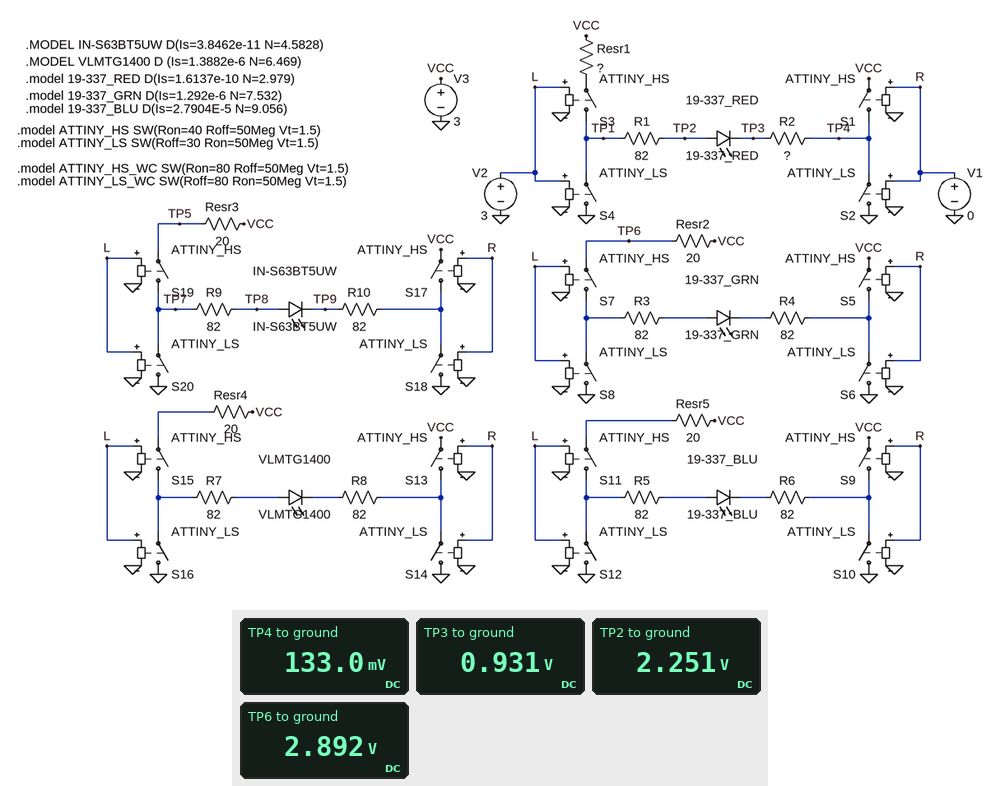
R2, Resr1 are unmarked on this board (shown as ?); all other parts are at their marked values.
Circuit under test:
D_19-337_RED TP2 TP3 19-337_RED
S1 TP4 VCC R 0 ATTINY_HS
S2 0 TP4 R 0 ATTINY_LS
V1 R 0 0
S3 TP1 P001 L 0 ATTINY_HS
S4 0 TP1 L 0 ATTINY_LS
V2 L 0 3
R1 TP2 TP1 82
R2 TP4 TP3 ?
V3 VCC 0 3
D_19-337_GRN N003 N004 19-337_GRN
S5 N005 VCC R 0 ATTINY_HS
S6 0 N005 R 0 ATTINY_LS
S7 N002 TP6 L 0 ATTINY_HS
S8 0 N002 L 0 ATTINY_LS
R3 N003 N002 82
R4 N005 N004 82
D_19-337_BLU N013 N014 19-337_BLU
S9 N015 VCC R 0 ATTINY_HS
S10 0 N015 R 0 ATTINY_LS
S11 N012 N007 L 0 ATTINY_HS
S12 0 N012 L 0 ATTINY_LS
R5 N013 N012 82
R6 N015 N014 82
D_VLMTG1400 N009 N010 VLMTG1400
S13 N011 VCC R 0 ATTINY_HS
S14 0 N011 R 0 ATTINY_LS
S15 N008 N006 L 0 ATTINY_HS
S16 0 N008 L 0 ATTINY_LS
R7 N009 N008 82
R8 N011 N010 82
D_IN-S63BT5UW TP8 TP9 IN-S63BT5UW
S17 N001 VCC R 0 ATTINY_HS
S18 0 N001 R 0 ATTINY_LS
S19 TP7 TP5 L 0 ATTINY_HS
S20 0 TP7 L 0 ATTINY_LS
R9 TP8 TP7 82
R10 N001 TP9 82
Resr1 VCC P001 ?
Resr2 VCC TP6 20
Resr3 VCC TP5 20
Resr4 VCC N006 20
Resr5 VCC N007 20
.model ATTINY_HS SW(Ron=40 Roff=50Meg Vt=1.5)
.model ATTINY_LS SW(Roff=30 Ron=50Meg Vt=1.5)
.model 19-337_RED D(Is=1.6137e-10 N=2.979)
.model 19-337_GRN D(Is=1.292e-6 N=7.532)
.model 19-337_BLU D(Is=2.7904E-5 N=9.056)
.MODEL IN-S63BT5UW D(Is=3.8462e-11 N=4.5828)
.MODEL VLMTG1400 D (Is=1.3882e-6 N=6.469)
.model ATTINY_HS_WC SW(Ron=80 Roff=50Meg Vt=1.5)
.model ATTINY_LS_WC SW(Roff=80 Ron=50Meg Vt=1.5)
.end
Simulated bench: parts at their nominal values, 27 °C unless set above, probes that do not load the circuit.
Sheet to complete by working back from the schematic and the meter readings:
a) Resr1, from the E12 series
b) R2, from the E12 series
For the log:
47 Ω
180 Ω
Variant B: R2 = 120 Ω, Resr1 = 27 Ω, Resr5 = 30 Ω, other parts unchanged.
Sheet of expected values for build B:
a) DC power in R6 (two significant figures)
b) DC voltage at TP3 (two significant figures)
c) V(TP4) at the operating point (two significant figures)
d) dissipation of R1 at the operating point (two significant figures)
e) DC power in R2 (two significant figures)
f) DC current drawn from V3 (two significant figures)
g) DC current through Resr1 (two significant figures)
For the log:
3.5 mW
830 mV
170 mV
2.5 mW
3.7 mW
27 mA
5.6 mA
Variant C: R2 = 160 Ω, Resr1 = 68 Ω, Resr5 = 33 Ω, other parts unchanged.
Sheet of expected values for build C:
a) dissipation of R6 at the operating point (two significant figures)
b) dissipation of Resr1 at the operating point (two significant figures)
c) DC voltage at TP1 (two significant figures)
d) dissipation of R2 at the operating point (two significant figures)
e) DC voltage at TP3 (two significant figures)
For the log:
3.4 mW
1.3 mW
2.5 V
3.1 mW
840 mV
